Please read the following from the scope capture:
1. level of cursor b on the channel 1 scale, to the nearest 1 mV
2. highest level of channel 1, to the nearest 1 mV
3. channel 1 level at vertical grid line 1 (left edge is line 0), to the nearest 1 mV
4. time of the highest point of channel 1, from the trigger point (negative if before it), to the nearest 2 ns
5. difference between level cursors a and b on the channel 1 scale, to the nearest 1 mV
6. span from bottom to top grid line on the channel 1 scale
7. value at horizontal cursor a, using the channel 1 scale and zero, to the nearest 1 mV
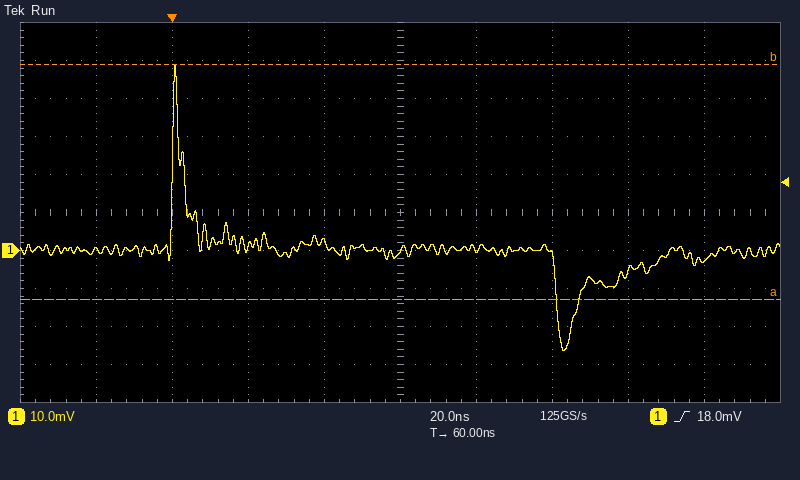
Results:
49 mV
49 mV
0 mV
0 ns
62 mV
100 mV
-13 mV
